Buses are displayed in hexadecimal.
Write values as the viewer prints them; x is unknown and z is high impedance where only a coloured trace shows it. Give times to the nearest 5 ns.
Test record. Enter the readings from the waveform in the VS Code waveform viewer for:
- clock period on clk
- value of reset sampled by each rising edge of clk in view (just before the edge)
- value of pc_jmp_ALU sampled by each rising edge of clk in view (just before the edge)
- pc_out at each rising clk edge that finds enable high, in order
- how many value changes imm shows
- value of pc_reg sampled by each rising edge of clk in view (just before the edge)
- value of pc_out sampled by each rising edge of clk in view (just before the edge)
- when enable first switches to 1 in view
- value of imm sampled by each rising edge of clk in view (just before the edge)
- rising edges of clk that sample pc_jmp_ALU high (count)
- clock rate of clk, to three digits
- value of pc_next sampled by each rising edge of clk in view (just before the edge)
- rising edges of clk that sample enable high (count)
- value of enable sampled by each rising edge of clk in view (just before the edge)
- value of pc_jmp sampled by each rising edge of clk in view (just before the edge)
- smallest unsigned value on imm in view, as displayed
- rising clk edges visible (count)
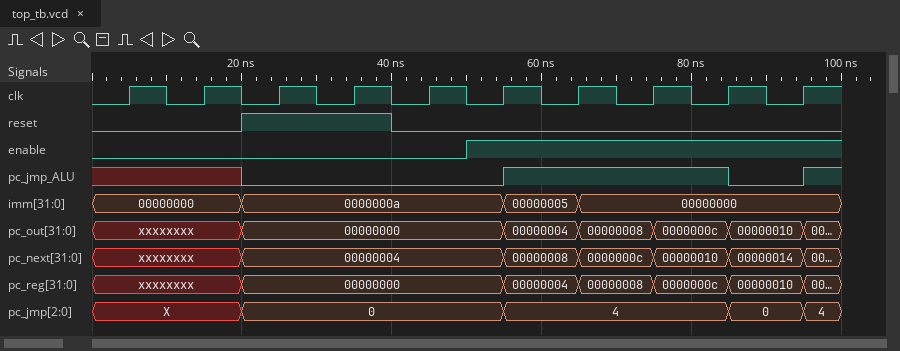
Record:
10 ns
0 0 1 1 0 0 0 0 0 0
x x 0 0 0 0 1 1 1 0
00000000, 00000004, 00000008, 0000000c, 00000010
3
xxxxxxxx, xxxxxxxx, 00000000, 00000000, 00000000, 00000000, 00000004, 00000008, 0000000c, 00000010
xxxxxxxx, xxxxxxxx, 00000000, 00000000, 00000000, 00000000, 00000004, 00000008, 0000000c, 00000010
50 ns
00000000, 00000000, 0000000a, 0000000a, 0000000a, 0000000a, 00000005, 00000000, 00000000, 00000000
3
100 MHz
xxxxxxxx, xxxxxxxx, 00000004, 00000004, 00000004, 00000004, 00000008, 0000000c, 00000010, 00000014
5
0 0 0 0 0 1 1 1 1 1
X, X, 0, 0, 0, 0, 4, 4, 4, 0
00000000
10
